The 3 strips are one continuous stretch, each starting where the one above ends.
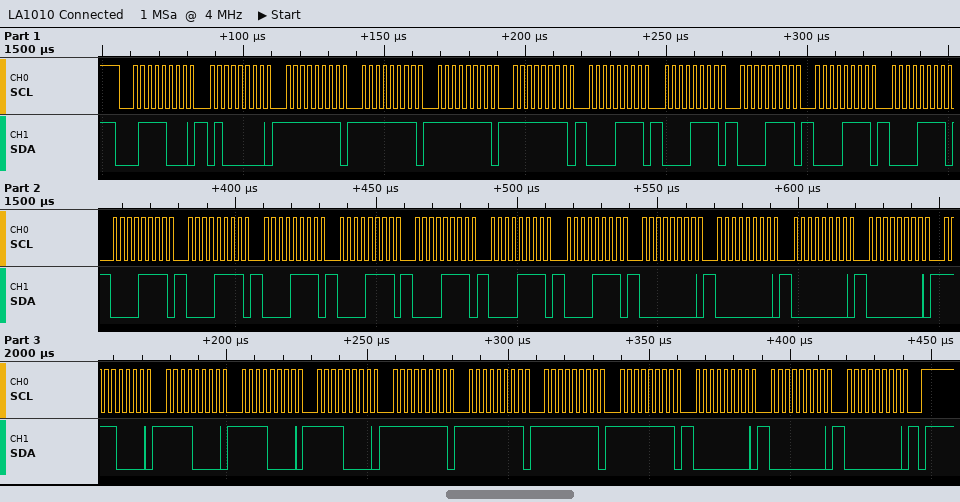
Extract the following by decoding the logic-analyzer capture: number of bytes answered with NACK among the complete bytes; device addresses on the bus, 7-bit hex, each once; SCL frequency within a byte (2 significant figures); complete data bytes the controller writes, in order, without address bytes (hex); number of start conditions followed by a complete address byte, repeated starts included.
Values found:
0
0x3C
400 kHz
40 FF FF FF FF 0F 0F 0F 0F 0F 0F 0F 0F 0F 0F 0F 0F 00 00 00 00 F0 F0 F0 F0 FF FF FF FF 00 00 00
1
